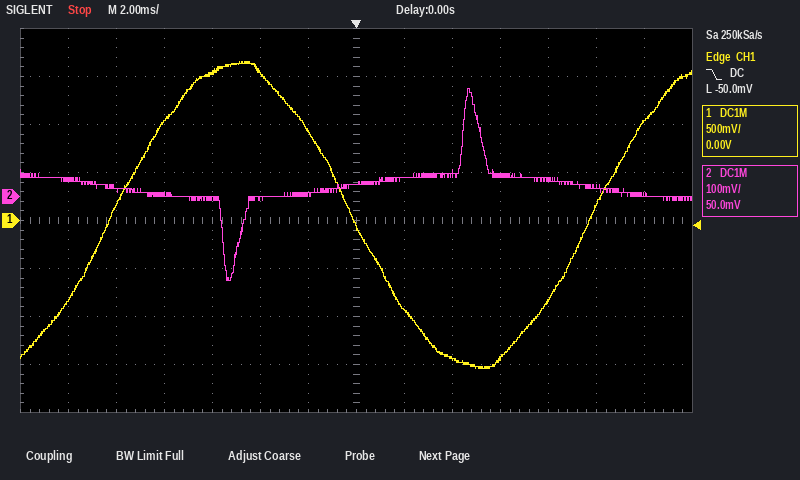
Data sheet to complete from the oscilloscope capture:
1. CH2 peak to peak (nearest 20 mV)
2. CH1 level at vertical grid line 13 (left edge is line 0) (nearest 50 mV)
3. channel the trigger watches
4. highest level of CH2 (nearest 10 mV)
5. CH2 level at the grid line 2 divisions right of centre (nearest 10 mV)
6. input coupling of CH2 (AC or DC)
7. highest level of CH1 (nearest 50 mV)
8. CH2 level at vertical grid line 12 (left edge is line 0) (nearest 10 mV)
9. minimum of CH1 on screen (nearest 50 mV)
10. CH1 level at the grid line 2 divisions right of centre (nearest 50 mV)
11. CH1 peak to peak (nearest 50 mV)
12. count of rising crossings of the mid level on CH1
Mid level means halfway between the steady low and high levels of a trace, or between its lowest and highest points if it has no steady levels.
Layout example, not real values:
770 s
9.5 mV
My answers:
400 mV
1.05 V
CH1
220 mV
50 mV
DC
1.65 V
20 mV
-1.55 V
-1.45 V
3.20 V
2
